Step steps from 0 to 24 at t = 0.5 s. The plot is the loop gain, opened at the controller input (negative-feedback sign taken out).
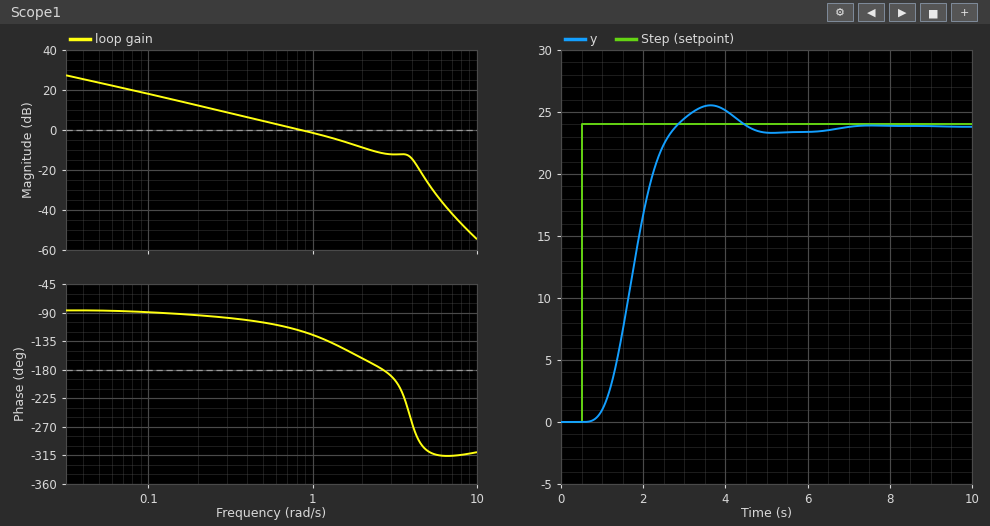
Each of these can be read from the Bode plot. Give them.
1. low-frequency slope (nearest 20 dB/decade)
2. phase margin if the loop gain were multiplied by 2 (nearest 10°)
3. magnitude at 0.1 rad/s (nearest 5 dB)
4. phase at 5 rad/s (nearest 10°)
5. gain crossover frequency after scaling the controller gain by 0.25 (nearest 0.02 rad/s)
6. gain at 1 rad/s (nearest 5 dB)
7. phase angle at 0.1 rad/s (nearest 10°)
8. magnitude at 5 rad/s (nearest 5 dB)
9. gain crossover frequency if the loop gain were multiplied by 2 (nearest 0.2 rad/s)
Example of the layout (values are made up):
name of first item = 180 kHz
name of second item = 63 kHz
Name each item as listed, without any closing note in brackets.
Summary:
low-frequency slope = -20 dB/decade
phase margin if the loop gain were multiplied by 2 = 30°
magnitude at 0.1 rad/s = 20 dB
phase at 5 rad/s = -310°
gain crossover frequency after scaling the controller gain by 0.25 = 0.20 rad/s
gain at 1 rad/s = 0 dB
phase angle at 0.1 rad/s = -90°
magnitude at 5 rad/s = -25 dB
gain crossover frequency if the loop gain were multiplied by 2 = 1.6 rad/s
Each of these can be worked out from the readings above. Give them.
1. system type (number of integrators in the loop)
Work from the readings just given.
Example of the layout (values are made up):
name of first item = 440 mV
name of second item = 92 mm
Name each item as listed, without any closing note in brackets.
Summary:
system type = 1
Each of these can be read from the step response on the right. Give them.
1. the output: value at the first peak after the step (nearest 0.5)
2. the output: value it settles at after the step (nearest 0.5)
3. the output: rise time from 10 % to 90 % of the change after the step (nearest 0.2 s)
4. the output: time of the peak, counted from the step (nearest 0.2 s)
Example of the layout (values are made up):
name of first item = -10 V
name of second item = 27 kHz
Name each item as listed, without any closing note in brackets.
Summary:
the output: value at the first peak after the step = 25.5
the output: value it settles at after the step = 24.0
the output: rise time from 10 % to 90 % of the change after the step = 1.2 s
the output: time of the peak, counted from the step = 3.2 s
